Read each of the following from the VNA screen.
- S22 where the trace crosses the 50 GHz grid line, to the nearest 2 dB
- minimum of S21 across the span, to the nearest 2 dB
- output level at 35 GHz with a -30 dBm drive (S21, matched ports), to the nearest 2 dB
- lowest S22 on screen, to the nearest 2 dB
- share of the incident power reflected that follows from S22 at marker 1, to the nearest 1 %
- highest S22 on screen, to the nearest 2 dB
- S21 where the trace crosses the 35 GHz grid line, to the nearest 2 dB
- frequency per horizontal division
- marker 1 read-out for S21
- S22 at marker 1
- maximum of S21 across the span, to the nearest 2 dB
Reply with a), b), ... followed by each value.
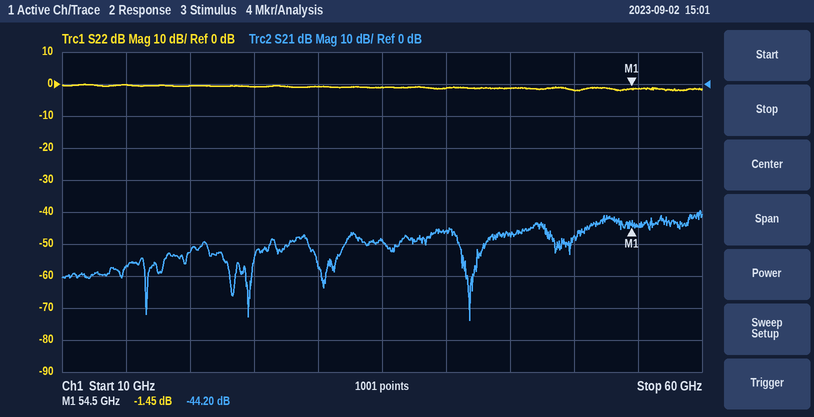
a) -2 dB
b) -74 dB
c) -78 dBm
d) -2 dB
e) 72 %
f) 0 dB
g) -48 dB
h) 5 GHz
i) -44.20 dB
j) -1.45 dB
k) -40 dB
